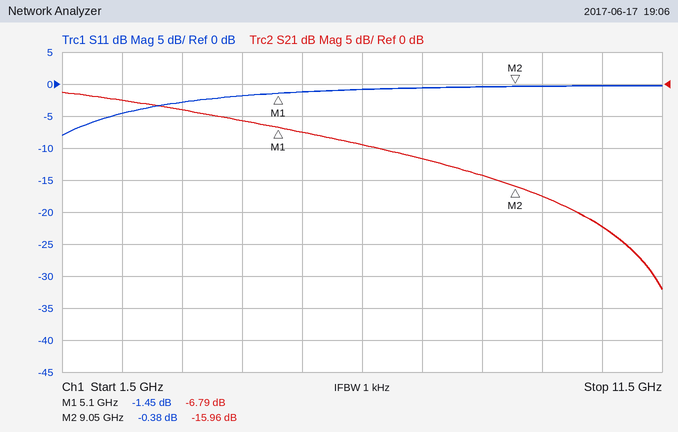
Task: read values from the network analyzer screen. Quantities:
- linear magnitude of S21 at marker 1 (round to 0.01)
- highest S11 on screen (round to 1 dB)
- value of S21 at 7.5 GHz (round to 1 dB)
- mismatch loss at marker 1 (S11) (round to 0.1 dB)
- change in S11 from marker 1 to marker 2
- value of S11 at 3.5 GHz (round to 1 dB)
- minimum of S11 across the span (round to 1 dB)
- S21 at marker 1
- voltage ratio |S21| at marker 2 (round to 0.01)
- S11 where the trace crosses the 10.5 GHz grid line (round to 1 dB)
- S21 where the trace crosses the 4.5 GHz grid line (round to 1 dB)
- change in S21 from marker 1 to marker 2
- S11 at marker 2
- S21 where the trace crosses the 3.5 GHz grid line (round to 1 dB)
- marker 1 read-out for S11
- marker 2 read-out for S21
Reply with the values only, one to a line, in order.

0.46
0 dB
-12 dB
5.5 dB
1.07 dB
-3 dB
-8 dB
-6.79 dB
0.16
0 dB
-6 dB
-9.17 dB
-0.38 dB
-4 dB
-1.45 dB
-15.96 dB
